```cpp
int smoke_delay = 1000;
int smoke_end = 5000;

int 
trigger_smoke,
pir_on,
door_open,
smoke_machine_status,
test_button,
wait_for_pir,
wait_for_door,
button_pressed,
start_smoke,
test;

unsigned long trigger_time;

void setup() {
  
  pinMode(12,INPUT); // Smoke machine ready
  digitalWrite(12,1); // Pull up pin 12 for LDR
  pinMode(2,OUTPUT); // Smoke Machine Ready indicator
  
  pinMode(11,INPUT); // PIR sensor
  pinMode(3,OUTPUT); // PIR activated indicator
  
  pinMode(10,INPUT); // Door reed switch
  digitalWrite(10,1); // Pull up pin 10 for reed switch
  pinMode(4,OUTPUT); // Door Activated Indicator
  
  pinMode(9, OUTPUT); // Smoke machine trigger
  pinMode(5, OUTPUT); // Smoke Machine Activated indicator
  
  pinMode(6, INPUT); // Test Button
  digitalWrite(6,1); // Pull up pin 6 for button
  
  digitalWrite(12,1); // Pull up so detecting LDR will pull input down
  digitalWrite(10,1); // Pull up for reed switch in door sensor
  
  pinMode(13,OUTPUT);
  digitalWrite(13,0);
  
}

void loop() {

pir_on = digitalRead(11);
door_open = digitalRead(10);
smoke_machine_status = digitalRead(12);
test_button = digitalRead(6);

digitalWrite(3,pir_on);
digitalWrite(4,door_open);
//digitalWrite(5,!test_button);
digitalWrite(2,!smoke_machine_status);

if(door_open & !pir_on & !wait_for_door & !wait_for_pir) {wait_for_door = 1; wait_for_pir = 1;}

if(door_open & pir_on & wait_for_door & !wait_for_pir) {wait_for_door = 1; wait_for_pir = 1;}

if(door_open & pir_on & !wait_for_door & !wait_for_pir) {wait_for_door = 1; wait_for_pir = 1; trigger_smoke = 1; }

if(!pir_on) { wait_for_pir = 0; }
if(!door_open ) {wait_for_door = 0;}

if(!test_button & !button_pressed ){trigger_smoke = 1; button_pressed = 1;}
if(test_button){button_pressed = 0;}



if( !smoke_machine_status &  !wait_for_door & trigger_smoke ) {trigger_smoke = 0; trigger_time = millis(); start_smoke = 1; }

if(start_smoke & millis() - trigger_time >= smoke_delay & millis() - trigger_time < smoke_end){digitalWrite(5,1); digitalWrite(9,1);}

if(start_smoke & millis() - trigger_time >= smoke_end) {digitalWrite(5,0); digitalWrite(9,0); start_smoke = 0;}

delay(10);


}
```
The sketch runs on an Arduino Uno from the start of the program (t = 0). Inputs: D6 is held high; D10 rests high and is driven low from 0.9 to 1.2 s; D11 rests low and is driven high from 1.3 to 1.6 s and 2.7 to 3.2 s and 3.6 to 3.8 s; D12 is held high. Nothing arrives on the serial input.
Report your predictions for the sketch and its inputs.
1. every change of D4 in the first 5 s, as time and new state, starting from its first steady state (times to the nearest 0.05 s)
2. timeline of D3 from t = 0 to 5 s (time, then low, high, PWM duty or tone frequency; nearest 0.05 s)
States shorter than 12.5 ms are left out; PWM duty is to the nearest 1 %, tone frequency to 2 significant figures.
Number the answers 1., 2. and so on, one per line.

1. 0 s high; 0.9 s low; 1.2 s high
2. 0 s low; 1.3 s high; 1.6 s low; 2.7 s high; 3.2 s low; 3.6 s high; 3.8 s low
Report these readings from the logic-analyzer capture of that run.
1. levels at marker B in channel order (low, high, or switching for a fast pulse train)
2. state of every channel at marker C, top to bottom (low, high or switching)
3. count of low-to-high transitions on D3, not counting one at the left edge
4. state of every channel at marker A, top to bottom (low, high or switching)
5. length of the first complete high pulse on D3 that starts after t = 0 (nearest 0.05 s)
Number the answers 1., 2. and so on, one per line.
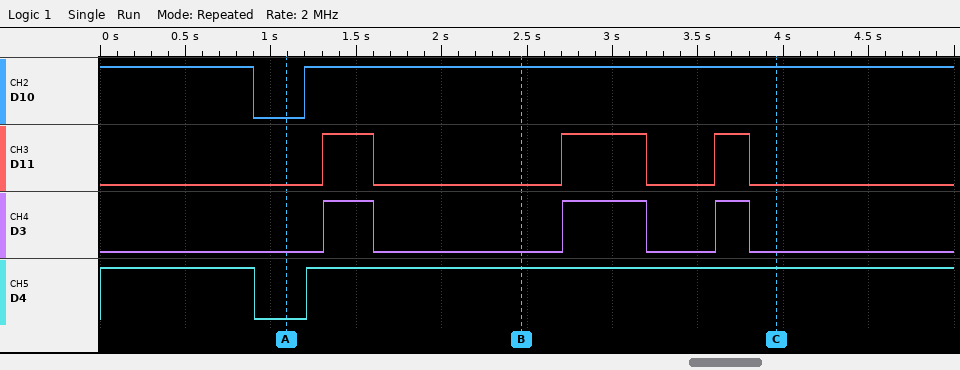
1. D10 high, D11 low, D3 low, D4 high
2. D10 high, D11 low, D3 low, D4 high
3. 3
4. D10 low, D11 low, D3 low, D4 low
5. 0.30 s
